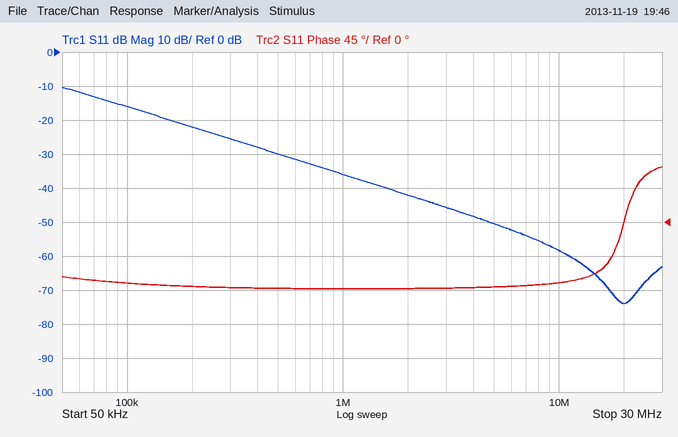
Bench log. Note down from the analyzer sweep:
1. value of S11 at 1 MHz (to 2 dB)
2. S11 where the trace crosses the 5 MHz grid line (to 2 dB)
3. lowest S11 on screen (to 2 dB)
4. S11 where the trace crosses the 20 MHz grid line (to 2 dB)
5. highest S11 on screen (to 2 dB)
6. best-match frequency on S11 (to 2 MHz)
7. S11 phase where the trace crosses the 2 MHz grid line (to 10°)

-36 dB
-50 dB
-74 dB
-74 dB
-10 dB
20 MHz
-90°
